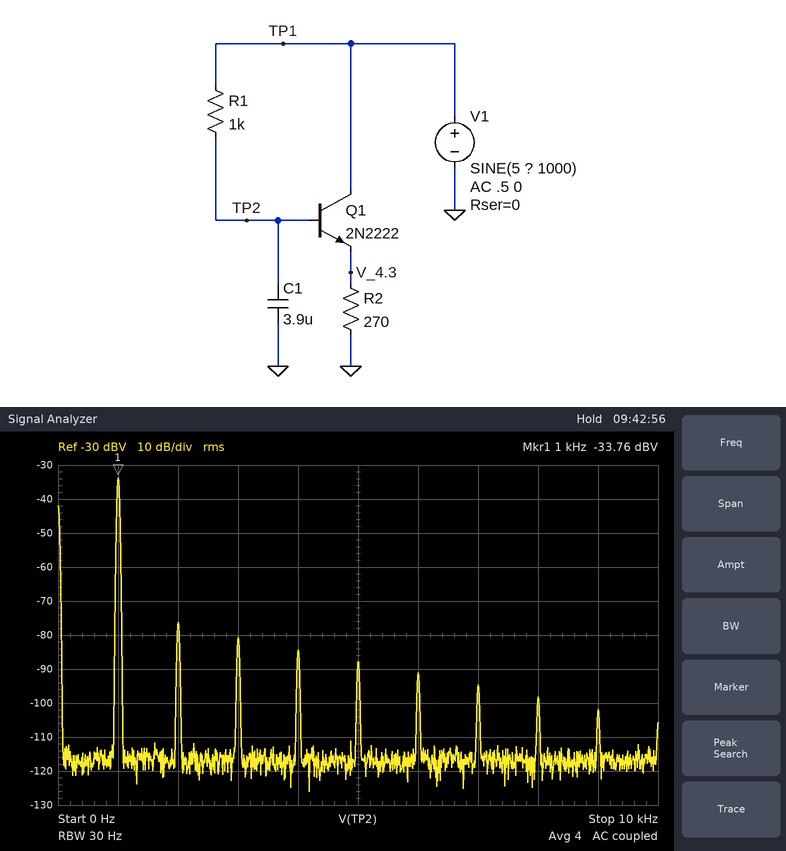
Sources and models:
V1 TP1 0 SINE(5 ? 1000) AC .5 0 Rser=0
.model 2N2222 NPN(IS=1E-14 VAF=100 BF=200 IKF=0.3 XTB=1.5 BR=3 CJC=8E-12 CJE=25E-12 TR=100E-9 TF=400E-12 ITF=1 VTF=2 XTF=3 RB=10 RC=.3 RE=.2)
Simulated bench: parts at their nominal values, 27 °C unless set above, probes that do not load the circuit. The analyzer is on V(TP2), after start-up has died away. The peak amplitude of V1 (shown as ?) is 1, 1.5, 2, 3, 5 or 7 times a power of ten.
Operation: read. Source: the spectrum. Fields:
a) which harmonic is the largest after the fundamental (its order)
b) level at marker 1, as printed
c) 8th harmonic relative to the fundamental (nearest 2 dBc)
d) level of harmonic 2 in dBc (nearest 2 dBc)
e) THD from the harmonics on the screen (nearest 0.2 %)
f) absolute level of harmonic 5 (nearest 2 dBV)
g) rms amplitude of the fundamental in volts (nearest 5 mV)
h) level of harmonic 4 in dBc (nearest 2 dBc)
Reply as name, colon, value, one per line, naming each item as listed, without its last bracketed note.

which harmonic is the largest after the fundamental: 2
level at marker 1, as printed: -33.76 dBV
8th harmonic relative to the fundamental: -64 dBc
level of harmonic 2 in dBc: -42 dBc
THD from the harmonics on the screen: 1.0 %
absolute level of harmonic 5: -88 dBV
rms amplitude of the fundamental in volts: 20 mV
level of harmonic 4 in dBc: -50 dBc
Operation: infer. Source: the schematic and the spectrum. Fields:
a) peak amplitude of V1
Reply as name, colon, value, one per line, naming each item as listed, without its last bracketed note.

peak amplitude of V1: 700 mV
